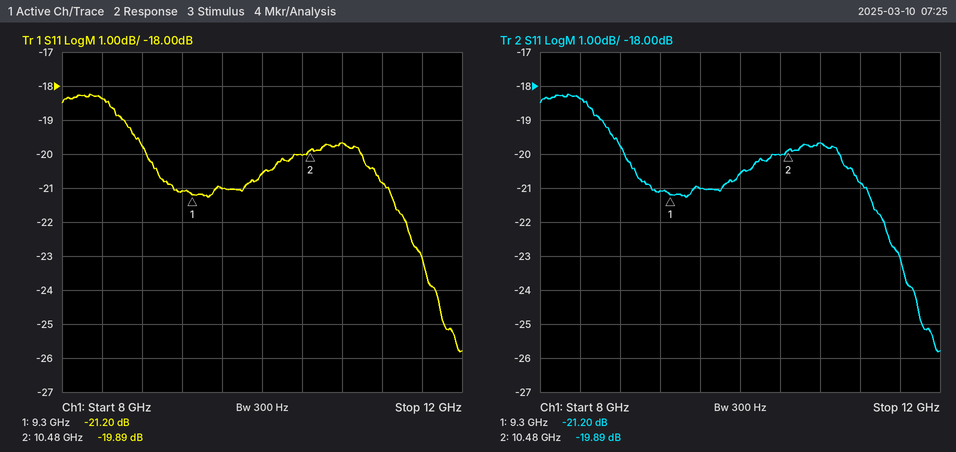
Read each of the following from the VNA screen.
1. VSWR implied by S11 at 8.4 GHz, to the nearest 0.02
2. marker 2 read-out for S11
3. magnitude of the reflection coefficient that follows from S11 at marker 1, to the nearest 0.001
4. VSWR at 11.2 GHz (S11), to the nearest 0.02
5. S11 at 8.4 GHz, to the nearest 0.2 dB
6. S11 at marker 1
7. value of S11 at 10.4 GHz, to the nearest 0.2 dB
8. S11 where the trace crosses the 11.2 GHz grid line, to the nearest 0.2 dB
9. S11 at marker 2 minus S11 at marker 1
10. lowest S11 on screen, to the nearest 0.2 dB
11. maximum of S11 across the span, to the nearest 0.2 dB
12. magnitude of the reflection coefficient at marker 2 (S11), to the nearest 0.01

1.28
-19.89 dB
0.087
1.20
-18.4 dB
-21.20 dB
-20.0 dB
-20.8 dB
1.31 dB
-25.8 dB
-18.2 dB
0.10
